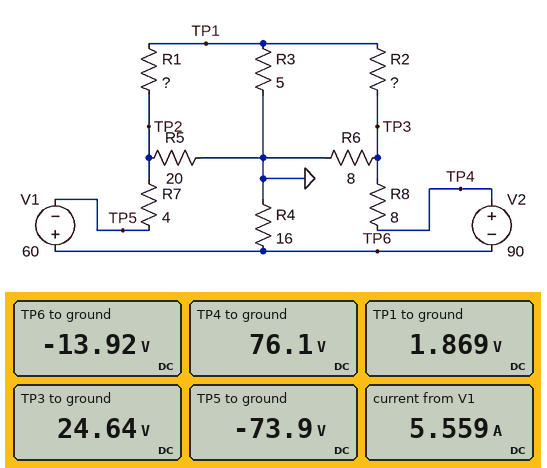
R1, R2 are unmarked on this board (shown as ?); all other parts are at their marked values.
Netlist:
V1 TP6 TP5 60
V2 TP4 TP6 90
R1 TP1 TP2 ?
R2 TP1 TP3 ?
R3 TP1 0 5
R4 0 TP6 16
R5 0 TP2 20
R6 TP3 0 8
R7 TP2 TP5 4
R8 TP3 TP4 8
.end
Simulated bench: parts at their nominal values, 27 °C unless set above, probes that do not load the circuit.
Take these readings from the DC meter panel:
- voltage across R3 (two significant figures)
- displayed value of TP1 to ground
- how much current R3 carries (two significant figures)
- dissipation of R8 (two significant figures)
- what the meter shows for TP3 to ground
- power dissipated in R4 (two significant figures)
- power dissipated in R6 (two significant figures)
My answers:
1.9 V
1.869 V
370 mA
330 W
24.64 V
12 W
76 W
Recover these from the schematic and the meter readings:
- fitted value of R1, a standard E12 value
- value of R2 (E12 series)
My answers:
18 Ω
6.8 Ω
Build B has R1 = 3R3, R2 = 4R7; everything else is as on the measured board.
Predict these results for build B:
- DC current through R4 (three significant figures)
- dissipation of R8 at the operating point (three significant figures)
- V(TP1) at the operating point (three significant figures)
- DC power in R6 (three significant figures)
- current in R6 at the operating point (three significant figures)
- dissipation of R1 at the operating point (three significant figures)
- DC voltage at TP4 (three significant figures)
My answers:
98.6 mA
564 W
-5.70 V
56.5 W
2.66 A
156 W
88.4 V
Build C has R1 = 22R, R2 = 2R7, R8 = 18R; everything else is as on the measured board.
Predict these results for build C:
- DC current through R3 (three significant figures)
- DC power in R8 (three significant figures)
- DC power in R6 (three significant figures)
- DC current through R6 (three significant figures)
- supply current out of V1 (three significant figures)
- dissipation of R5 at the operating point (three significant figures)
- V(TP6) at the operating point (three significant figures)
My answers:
750 mA
338 W
16.7 W
1.44 A
4.30 A
93.6 W
-482 mV
